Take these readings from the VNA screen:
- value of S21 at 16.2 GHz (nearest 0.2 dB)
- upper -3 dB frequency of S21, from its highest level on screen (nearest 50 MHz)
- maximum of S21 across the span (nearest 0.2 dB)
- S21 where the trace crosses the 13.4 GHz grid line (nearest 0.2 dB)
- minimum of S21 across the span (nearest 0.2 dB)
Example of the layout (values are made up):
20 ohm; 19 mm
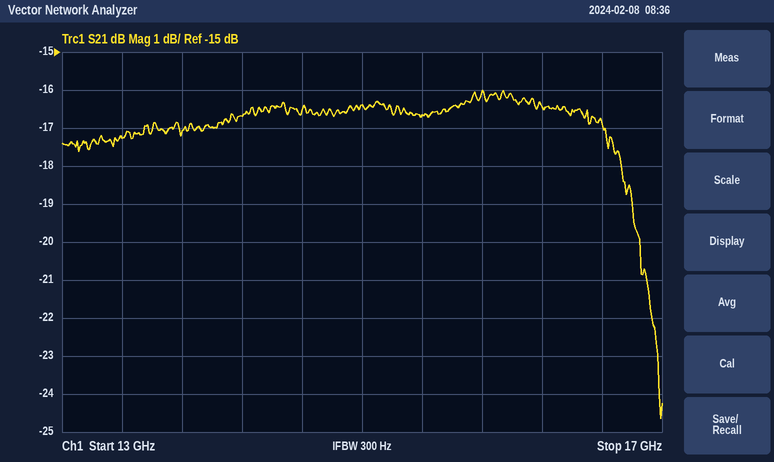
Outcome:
-16.4 dB; 16.80 GHz; -16.0 dB; -17.2 dB; -24.6 dB
